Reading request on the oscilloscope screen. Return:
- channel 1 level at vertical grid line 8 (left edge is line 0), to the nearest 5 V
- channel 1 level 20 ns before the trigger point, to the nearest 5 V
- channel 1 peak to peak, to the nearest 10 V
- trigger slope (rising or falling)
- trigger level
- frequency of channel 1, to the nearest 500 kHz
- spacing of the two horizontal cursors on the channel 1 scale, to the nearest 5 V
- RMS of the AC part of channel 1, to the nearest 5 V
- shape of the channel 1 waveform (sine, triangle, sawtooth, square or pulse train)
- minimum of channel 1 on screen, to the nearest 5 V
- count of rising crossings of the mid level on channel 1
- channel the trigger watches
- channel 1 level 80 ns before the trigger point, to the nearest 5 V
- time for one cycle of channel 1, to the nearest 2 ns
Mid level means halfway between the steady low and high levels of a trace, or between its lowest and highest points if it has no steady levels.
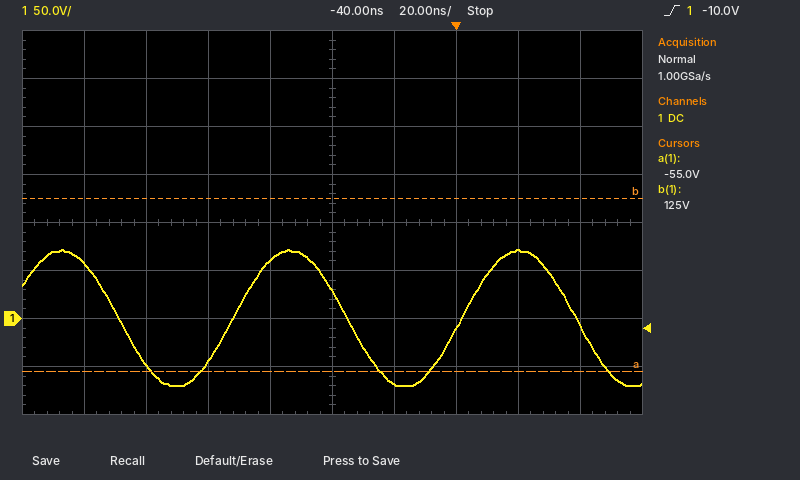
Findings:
70 V
-70 V
140 V
rising
-10.0 V
13.5 MHz
180 V
50 V
sine
-70 V
2
channel 1
-45 V
74 ns
